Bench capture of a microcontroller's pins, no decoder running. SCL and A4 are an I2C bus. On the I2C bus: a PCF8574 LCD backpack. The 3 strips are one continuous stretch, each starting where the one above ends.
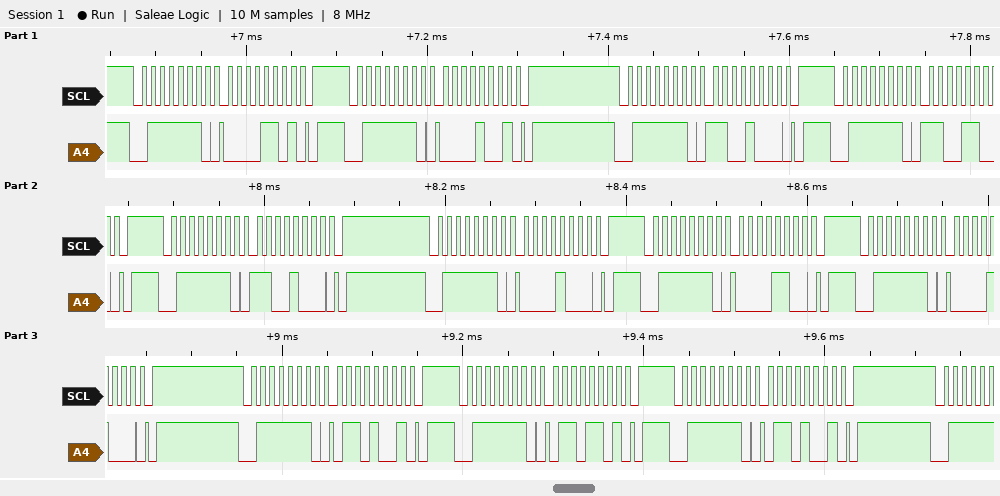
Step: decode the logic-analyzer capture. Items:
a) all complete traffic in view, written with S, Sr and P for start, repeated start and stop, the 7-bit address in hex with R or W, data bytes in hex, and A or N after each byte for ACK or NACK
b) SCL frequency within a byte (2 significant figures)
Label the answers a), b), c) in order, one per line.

a) S 3FW A 0D A P S 3FW A 09 A P S 3FW A C8 A P S 3FW A CC A P S 3FW A C8 A P S 3FW A 08 A P S 3FW A 0C A P S 3FW A 08 A P S 3FW A 69 A P S 3FW A 6D A P S 3FW A 69 A P
b) 100 kHz
